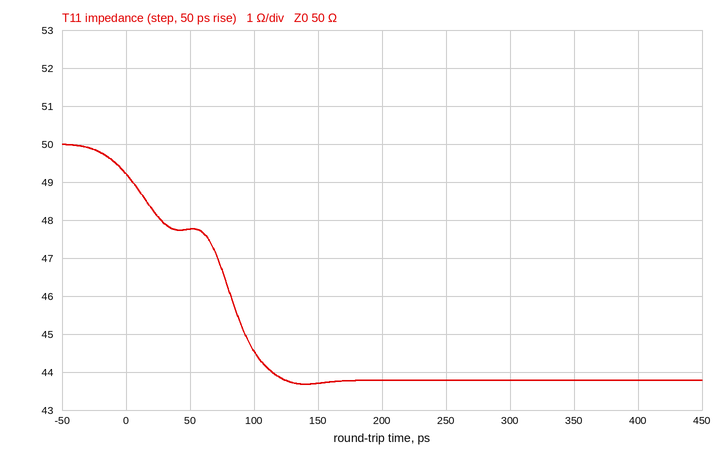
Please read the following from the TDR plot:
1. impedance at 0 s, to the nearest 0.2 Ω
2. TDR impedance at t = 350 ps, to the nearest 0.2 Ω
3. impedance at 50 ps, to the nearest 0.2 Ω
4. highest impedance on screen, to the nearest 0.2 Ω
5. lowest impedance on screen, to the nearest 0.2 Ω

49.2 Ω
43.8 Ω
47.8 Ω
50.0 Ω
43.6 Ω
